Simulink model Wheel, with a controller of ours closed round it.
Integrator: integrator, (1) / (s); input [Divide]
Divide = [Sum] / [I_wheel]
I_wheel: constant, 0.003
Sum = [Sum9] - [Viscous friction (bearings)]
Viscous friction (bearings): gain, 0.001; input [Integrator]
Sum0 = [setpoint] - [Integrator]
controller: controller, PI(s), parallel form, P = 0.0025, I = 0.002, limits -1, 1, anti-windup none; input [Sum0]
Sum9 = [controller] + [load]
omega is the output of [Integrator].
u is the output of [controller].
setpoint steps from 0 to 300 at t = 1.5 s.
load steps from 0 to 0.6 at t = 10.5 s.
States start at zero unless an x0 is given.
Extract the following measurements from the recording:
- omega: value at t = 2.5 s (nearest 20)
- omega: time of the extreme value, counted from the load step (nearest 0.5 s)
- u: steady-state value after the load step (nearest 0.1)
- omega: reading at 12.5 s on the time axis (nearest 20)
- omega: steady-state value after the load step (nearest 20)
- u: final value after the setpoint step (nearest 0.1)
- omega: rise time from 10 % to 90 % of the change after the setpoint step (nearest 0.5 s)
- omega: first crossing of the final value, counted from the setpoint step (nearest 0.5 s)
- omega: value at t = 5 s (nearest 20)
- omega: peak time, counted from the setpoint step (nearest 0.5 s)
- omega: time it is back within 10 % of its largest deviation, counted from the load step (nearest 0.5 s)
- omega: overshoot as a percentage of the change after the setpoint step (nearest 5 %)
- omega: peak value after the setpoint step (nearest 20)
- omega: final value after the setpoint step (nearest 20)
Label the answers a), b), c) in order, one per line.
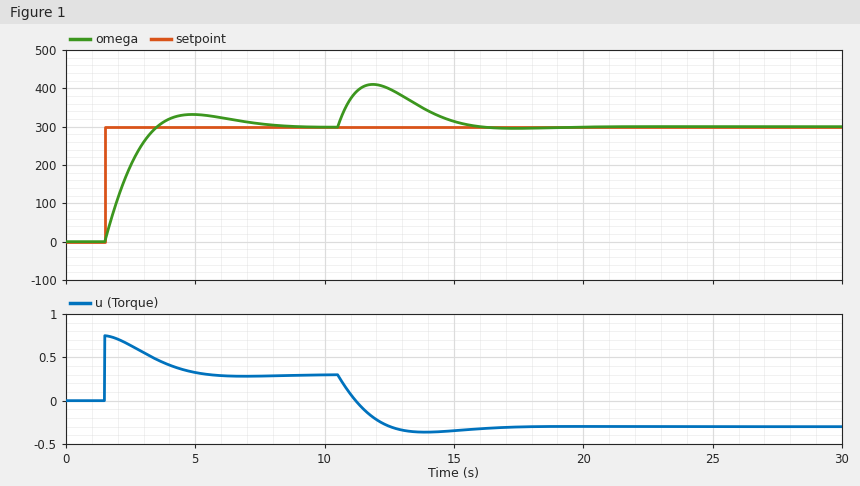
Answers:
a) 200
b) 1.5 s
c) -0.3
d) 400
e) 300
f) 0.3
g) 1.5 s
h) 2.0 s
i) 340
j) 3.5 s
k) 4.5 s
l) 10 %
m) 340
n) 300
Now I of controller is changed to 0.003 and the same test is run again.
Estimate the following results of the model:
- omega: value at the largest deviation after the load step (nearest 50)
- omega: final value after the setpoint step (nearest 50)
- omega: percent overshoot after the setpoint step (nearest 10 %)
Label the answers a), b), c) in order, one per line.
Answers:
a) 400
b) 300
c) 20 %
